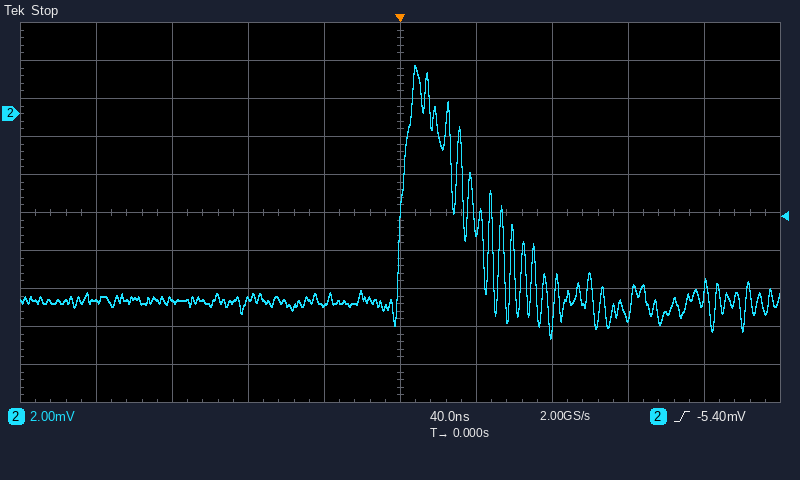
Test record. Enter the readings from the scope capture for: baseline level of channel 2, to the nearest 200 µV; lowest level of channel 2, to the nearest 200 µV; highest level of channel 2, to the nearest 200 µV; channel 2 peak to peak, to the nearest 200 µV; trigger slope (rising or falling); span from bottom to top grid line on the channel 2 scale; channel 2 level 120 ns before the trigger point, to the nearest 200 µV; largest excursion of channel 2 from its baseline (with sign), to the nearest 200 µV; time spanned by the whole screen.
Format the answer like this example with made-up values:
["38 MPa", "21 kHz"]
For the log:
["-9.8 mV", "-11.8 mV", "2.6 mV", "14.4 mV", "rising", "20 mV", "-9.8 mV", "+12.4 mV", "400 ns"]
